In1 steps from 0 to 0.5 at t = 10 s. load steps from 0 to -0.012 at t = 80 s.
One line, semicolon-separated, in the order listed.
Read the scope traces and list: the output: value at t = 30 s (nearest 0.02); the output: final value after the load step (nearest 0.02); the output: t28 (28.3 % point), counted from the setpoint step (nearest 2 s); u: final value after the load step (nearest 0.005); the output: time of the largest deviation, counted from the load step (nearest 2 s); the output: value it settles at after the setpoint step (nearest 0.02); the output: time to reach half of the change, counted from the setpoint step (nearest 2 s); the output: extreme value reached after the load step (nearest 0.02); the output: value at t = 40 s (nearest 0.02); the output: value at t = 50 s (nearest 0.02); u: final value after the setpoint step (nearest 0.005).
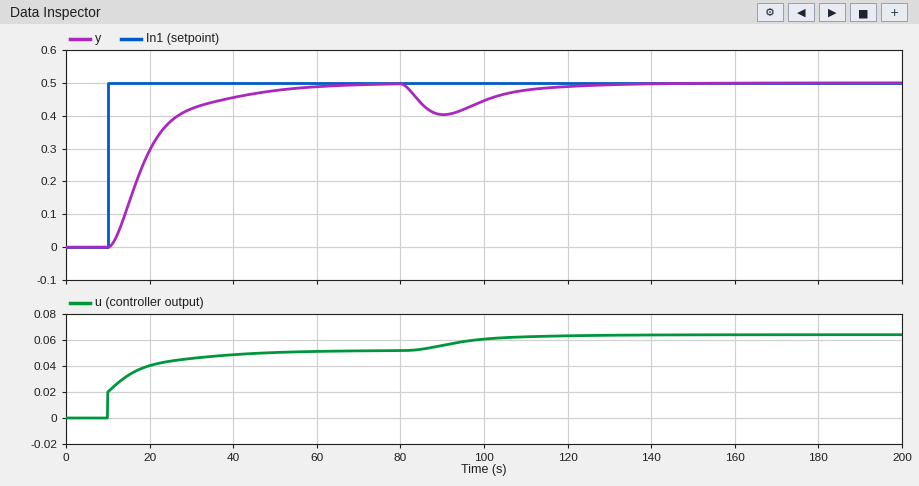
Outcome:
0.42; 0.50; 6 s; 0.065; 10 s; 0.50; 8 s; 0.40; 0.46; 0.48; 0.050
